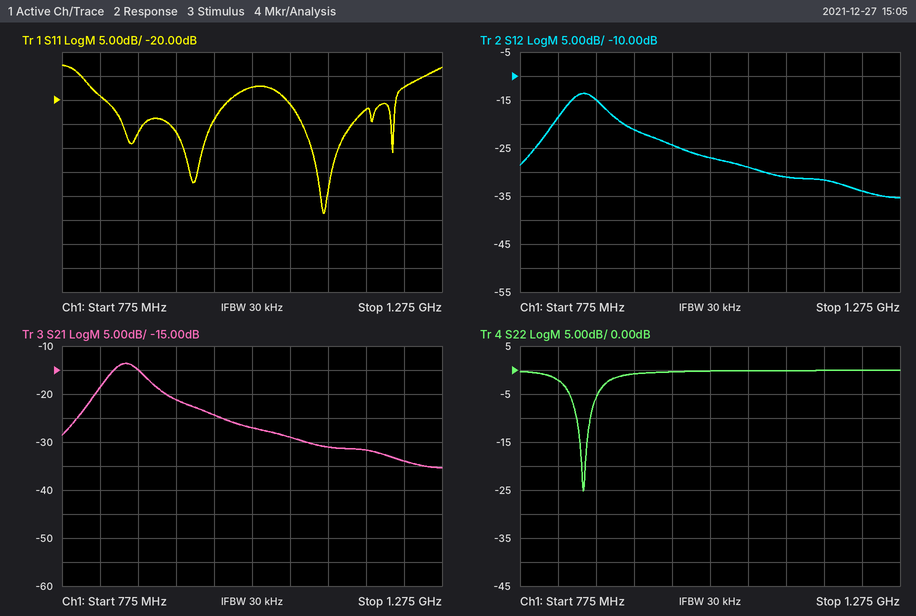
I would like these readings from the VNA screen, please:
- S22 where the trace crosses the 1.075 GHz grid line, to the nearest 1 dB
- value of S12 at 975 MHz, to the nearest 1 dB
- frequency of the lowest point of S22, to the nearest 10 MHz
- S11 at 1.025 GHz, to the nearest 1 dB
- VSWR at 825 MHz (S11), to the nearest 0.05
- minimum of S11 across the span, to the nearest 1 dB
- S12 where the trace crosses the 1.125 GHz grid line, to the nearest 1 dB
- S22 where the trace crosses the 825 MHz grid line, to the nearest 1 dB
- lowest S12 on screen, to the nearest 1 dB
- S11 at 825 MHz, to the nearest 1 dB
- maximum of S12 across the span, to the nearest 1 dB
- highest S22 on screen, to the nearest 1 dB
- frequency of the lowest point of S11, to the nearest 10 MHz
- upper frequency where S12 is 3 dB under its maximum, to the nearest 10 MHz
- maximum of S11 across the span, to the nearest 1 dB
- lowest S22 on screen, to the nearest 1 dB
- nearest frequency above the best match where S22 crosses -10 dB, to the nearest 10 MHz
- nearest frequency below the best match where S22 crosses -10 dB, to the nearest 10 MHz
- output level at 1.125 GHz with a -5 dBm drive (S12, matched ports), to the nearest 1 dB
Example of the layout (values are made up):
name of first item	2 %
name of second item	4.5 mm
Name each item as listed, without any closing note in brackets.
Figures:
S22 where the trace crosses the 1.075 GHz grid line, to the nearest 1 dB	0 dB
value of S12 at 975 MHz, to the nearest 1 dB	-24 dB
frequency of the lowest point of S22, to the nearest 10 MHz	860 MHz
S11 at 1.025 GHz, to the nearest 1 dB	-17 dB
VSWR at 825 MHz (S11), to the nearest 0.05	1.25
minimum of S11 across the span, to the nearest 1 dB	-44 dB
S12 where the trace crosses the 1.125 GHz grid line, to the nearest 1 dB	-31 dB
S22 where the trace crosses the 825 MHz grid line, to the nearest 1 dB	-2 dB
lowest S12 on screen, to the nearest 1 dB	-35 dB
S11 at 825 MHz, to the nearest 1 dB	-19 dB
maximum of S12 across the span, to the nearest 1 dB	-14 dB
highest S22 on screen, to the nearest 1 dB	0 dB
frequency of the lowest point of S11, to the nearest 10 MHz	1.12 GHz
upper frequency where S12 is 3 dB under its maximum, to the nearest 10 MHz	890 MHz
maximum of S11 across the span, to the nearest 1 dB	-13 dB
lowest S22 on screen, to the nearest 1 dB	-25 dB
nearest frequency above the best match where S22 crosses -10 dB, to the nearest 10 MHz	870 MHz
nearest frequency below the best match where S22 crosses -10 dB, to the nearest 10 MHz	850 MHz
output level at 1.125 GHz with a -5 dBm drive (S12, matched ports), to the nearest 1 dB	-36 dBm
